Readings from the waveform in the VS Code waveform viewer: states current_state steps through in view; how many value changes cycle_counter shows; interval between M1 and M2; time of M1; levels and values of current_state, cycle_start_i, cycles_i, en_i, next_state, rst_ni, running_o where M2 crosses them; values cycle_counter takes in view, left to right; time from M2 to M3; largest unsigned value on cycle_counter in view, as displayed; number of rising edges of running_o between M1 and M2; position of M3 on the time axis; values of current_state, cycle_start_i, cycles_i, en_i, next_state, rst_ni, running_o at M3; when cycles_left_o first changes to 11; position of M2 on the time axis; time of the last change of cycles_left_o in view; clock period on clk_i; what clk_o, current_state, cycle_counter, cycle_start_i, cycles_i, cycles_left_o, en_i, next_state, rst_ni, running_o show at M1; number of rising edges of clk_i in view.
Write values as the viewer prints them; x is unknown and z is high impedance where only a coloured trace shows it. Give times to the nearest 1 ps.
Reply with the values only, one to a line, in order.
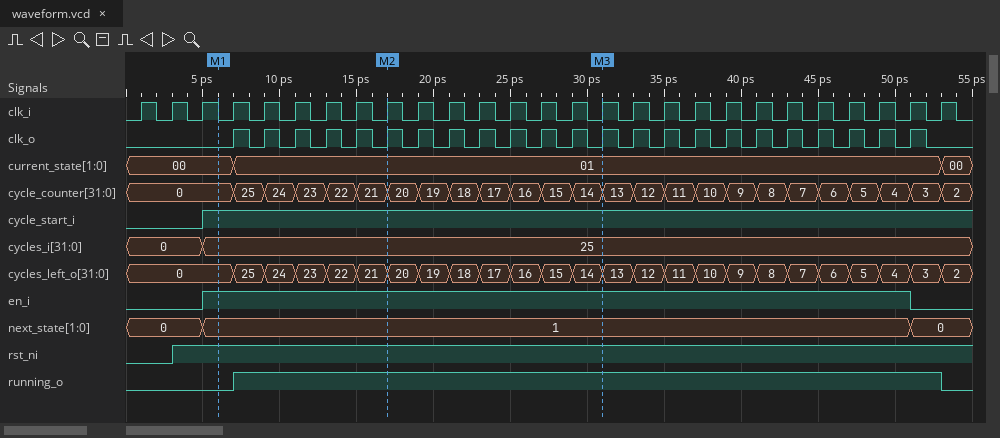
00, 01, 00
24
11 ps
6 ps
current_state=01, cycle_start_i=1, cycles_i=25, en_i=1, next_state=1, rst_ni=1, running_o=1
0, 25, 24, 23, 22, 21, 20, 19, 18, 17, 16, 15, 14, 13, 12, 11, 10, 9, 8, 7, 6, 5, 4, 3, 2
14 ps
25
1
31 ps
current_state=01, cycle_start_i=1, cycles_i=25, en_i=1, next_state=1, rst_ni=1, running_o=1
35 ps
17 ps
53 ps
2 ps
clk_o=0, current_state=00, cycle_counter=0, cycle_start_i=1, cycles_i=25, cycles_left_o=0, en_i=1, next_state=1, rst_ni=1, running_o=0
27
